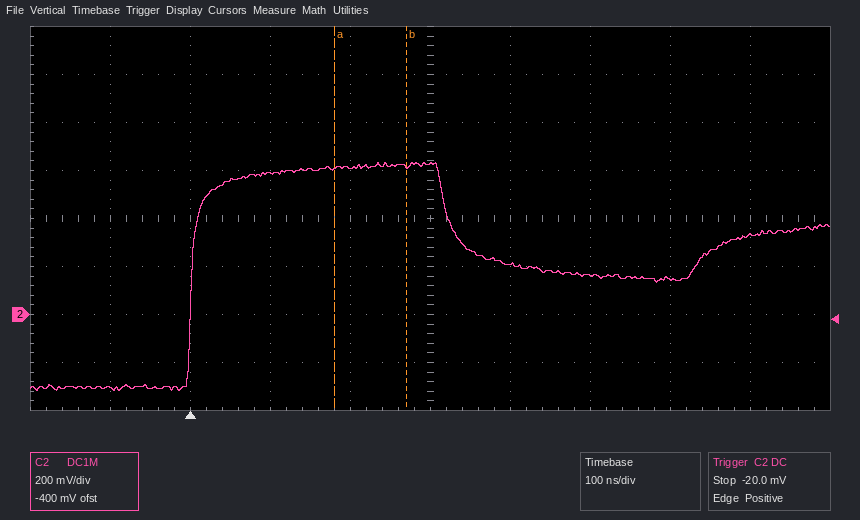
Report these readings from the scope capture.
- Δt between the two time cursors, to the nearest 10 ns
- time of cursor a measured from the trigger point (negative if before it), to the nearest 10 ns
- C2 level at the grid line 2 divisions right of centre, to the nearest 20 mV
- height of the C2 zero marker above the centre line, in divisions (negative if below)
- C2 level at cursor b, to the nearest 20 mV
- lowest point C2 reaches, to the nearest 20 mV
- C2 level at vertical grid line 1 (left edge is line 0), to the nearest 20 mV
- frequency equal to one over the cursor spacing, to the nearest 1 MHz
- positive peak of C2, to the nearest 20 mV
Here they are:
90 ns
+180 ns
160 mV
-2.0 div
620 mV
-320 mV
-300 mV
11 MHz
640 mV
